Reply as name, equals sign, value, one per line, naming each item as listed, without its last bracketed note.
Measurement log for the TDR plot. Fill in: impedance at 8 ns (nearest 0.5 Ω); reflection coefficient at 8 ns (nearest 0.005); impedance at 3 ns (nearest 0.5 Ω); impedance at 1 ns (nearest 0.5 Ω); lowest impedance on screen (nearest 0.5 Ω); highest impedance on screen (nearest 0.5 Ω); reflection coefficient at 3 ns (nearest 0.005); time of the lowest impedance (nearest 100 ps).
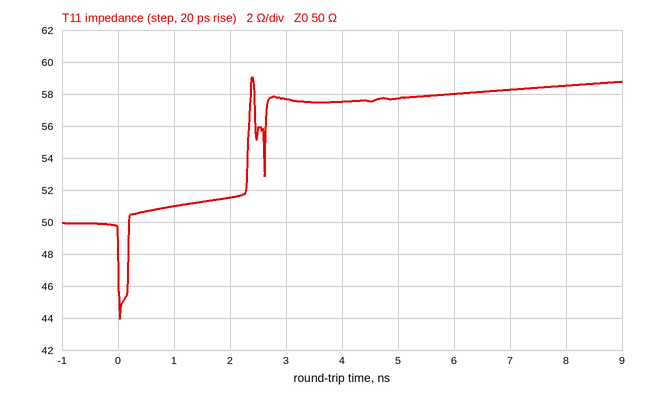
impedance at 8 ns = 58.5 Ω
reflection coefficient at 8 ns = +0.080
impedance at 3 ns = 57.5 Ω
impedance at 1 ns = 51.0 Ω
lowest impedance on screen = 44.0 Ω
highest impedance on screen = 59.0 Ω
reflection coefficient at 3 ns = +0.070
time of the lowest impedance = 0.0 ns
